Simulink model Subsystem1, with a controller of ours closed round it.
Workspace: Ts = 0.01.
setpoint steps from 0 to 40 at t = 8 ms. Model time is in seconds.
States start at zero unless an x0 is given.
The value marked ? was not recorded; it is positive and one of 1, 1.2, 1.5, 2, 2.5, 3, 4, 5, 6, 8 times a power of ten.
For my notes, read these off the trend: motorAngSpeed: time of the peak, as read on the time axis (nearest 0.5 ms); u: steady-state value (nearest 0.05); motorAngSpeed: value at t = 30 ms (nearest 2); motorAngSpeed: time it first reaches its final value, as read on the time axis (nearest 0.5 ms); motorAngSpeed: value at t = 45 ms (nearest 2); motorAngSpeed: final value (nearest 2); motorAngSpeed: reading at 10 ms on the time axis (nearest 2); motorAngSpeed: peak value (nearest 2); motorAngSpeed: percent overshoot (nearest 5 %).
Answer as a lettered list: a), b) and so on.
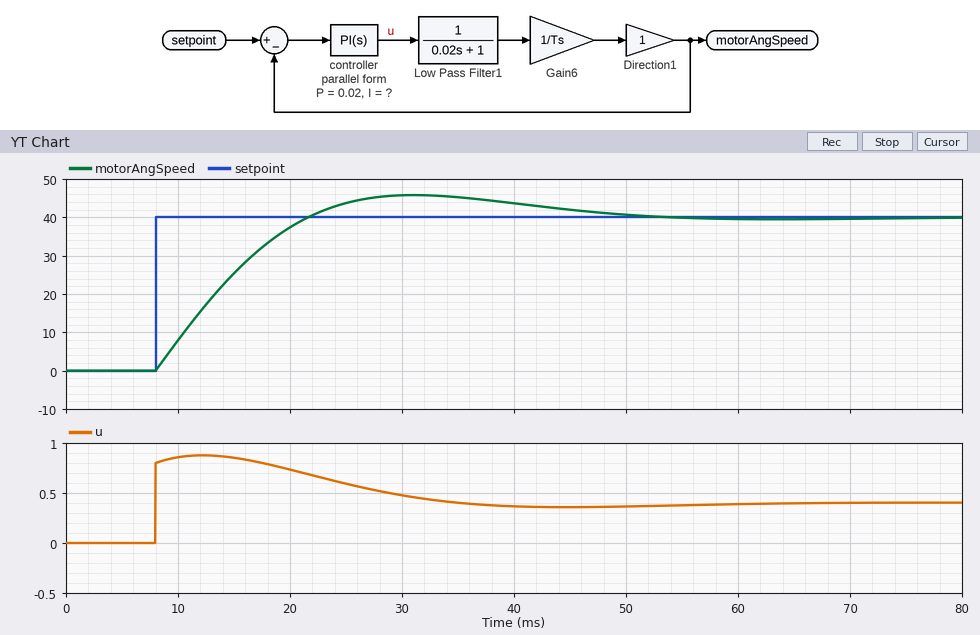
a) 31.0 ms
b) 0.40
c) 46
d) 21.5 ms
e) 42
f) 40
g) 8
h) 46
i) 15 %
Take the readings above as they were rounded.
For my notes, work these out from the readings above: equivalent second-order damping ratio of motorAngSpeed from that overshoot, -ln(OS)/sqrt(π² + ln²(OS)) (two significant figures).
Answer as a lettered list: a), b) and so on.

a) 0.52
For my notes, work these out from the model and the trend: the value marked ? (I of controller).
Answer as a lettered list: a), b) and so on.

a) 3
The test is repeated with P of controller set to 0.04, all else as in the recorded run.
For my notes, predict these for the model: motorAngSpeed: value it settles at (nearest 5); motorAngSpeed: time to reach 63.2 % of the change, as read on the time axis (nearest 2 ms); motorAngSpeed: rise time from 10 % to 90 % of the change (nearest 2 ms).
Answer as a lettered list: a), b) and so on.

a) 40
b) 12 ms
c) 8 ms
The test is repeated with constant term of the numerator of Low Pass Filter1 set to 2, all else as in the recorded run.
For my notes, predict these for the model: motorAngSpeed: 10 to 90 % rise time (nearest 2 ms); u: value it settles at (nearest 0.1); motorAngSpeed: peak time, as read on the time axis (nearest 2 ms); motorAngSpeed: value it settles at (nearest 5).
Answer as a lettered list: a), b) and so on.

a) 6 ms
b) 0.2
c) 22 ms
d) 40
